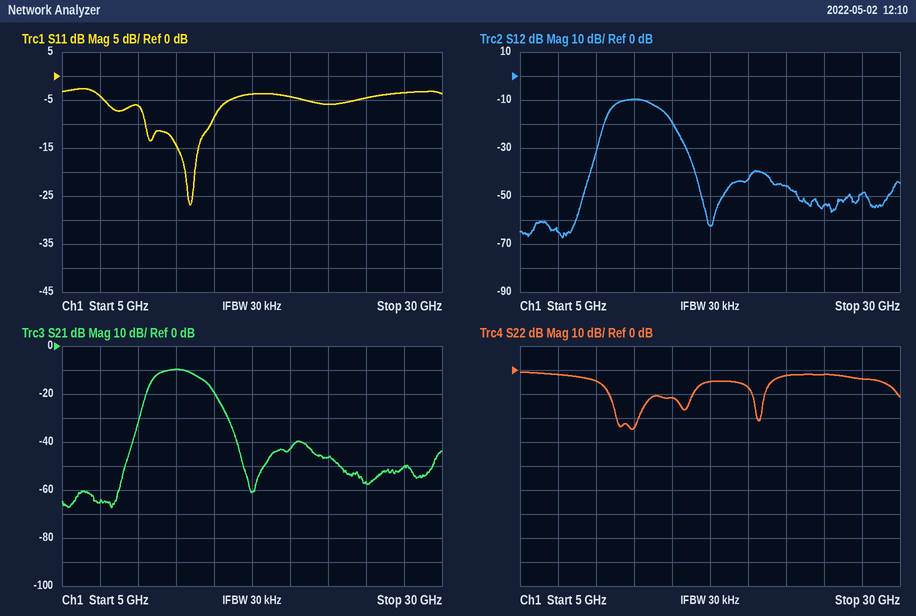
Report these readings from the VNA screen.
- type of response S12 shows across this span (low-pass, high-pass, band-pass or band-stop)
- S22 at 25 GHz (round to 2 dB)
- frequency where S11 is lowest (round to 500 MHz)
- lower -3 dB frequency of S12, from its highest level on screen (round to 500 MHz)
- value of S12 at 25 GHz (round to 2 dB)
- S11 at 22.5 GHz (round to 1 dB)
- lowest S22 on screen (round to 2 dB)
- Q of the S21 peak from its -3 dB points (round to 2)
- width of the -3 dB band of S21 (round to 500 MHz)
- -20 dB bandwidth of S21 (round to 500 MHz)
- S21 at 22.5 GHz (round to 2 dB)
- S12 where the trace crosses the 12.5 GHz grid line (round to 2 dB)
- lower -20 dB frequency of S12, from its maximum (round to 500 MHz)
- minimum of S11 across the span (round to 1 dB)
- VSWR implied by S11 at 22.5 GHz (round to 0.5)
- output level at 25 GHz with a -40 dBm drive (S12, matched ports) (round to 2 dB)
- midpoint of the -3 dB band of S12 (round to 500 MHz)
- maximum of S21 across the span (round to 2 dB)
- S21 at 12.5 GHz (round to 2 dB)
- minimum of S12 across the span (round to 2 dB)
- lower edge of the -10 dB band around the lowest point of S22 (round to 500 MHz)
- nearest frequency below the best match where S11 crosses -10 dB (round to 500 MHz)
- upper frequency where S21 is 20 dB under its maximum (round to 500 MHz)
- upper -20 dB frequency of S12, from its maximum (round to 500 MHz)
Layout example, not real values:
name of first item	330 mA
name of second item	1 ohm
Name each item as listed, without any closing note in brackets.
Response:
type of response S12 shows across this span	band-pass
S22 at 25 GHz	-2 dB
frequency where S11 is lowest	13.5 GHz
lower -3 dB frequency of S12, from its highest level on screen	11.0 GHz
value of S12 at 25 GHz	-54 dB
S11 at 22.5 GHz	-6 dB
lowest S22 on screen	-24 dB
Q of the S21 peak from its -3 dB points	4
width of the -3 dB band of S21	3.0 GHz
-20 dB bandwidth of S21	6.0 GHz
S21 at 22.5 GHz	-46 dB
S12 where the trace crosses the 12.5 GHz grid line	-10 dB
lower -20 dB frequency of S12, from its maximum	10.0 GHz
minimum of S11 across the span	-27 dB
VSWR implied by S11 at 22.5 GHz	3.0
output level at 25 GHz with a -40 dBm drive (S12, matched ports)	-94 dBm
midpoint of the -3 dB band of S12	12.5 GHz
maximum of S21 across the span	-10 dB
S21 at 12.5 GHz	-10 dB
minimum of S12 across the span	-68 dB
lower edge of the -10 dB band around the lowest point of S22	11.0 GHz
nearest frequency below the best match where S11 crosses -10 dB	10.5 GHz
upper frequency where S21 is 20 dB under its maximum	16.0 GHz
upper -20 dB frequency of S12, from its maximum	16.0 GHz
